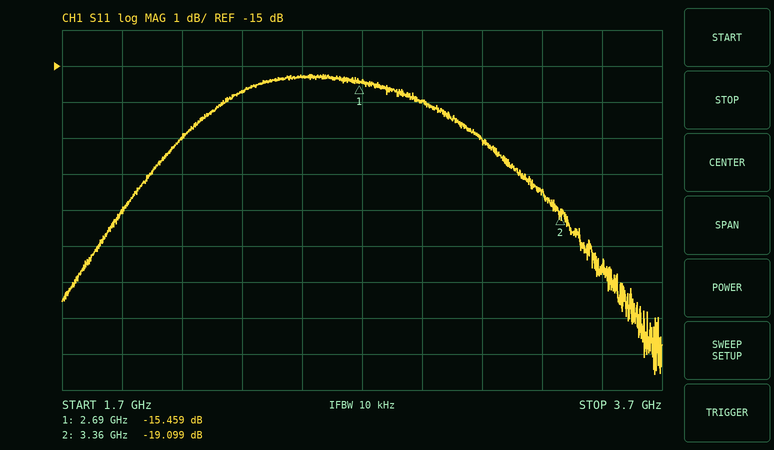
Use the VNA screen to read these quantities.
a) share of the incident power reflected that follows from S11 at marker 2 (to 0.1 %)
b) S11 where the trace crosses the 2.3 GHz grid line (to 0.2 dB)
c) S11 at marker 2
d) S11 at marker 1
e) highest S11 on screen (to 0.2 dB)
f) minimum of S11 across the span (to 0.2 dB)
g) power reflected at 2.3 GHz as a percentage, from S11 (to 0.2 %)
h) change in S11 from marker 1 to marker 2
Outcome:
1.2 %
-15.8 dB
-19.099 dB
-15.459 dB
-15.2 dB
-23.6 dB
2.6 %
-3.640 dB
